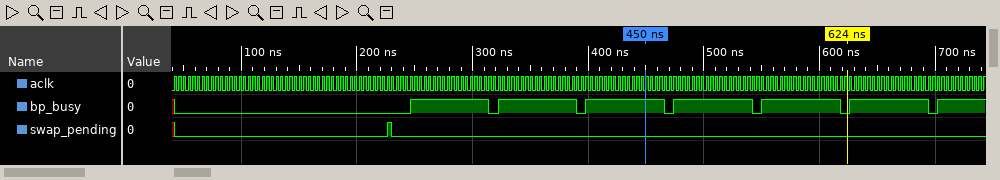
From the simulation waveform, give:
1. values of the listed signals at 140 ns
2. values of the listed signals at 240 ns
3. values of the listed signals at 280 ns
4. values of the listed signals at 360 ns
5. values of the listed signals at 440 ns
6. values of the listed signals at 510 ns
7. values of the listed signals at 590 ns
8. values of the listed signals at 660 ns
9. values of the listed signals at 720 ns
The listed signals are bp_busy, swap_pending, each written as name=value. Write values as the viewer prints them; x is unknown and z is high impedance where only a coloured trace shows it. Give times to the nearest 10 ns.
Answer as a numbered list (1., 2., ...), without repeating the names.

1. bp_busy=0, swap_pending=0
2. bp_busy=0, swap_pending=0
3. bp_busy=1, swap_pending=0
4. bp_busy=1, swap_pending=0
5. bp_busy=1, swap_pending=0
6. bp_busy=1, swap_pending=0
7. bp_busy=1, swap_pending=0
8. bp_busy=1, swap_pending=0
9. bp_busy=1, swap_pending=0
